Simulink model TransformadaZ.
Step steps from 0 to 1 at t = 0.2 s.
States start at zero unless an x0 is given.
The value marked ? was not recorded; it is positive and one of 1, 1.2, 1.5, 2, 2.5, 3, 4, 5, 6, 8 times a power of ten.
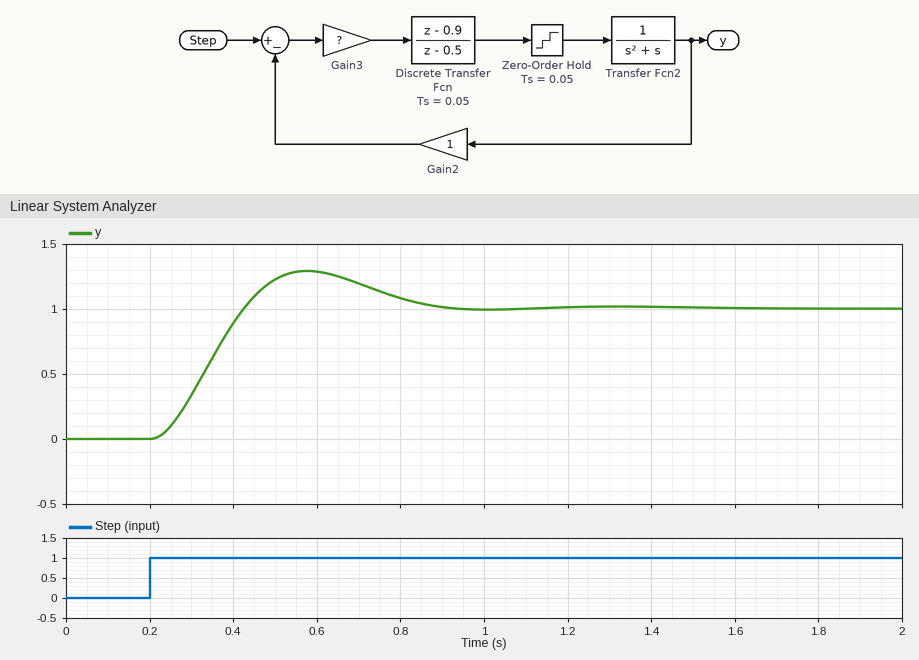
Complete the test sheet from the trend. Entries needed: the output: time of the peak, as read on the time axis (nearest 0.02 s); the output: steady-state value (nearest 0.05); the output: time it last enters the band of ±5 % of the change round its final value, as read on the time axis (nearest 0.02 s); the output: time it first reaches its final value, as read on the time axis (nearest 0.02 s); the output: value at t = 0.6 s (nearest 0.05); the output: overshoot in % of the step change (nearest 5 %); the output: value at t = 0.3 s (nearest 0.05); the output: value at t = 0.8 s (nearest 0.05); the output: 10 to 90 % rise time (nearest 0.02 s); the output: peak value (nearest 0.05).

0.58 s
1.00
0.84 s
0.42 s
1.30
30 %
0.35
1.10
0.16 s
1.30
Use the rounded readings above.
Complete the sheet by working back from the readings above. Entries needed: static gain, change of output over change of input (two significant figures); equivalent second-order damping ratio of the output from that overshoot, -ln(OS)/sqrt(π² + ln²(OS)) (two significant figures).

1.0
0.36
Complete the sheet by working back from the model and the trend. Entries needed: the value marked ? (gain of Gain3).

80
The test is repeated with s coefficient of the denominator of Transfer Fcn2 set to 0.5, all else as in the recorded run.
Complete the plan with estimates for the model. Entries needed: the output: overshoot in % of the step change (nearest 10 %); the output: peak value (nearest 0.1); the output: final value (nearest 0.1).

40 %
1.4
1.0
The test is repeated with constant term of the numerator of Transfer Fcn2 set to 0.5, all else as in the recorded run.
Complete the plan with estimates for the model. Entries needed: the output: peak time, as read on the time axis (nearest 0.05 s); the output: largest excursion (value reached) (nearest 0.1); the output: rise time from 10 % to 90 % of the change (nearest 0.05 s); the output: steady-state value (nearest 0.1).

0.90 s
1.2
0.30 s
1.0
